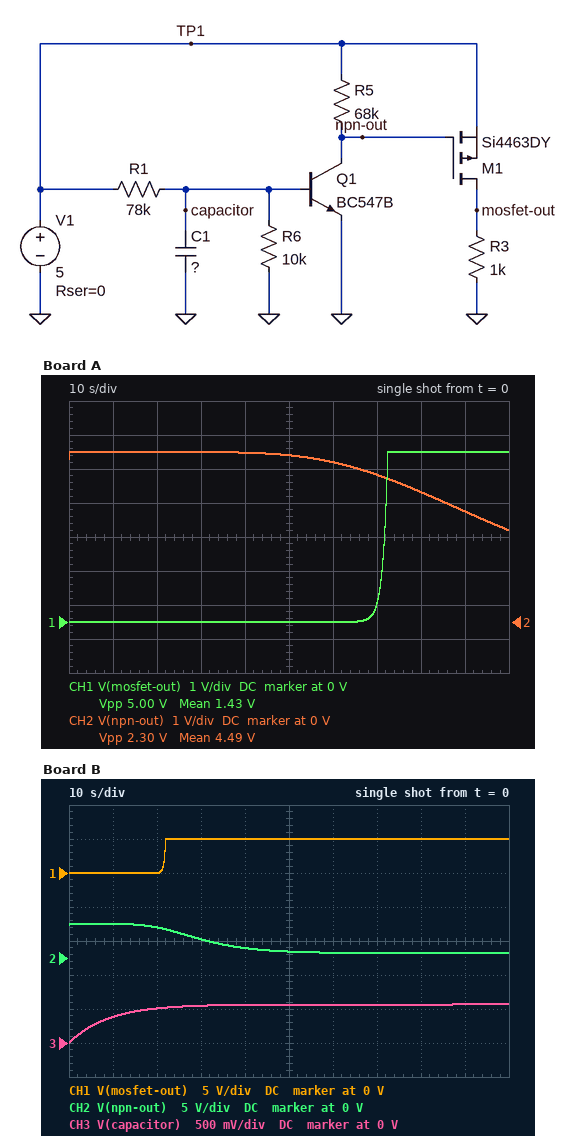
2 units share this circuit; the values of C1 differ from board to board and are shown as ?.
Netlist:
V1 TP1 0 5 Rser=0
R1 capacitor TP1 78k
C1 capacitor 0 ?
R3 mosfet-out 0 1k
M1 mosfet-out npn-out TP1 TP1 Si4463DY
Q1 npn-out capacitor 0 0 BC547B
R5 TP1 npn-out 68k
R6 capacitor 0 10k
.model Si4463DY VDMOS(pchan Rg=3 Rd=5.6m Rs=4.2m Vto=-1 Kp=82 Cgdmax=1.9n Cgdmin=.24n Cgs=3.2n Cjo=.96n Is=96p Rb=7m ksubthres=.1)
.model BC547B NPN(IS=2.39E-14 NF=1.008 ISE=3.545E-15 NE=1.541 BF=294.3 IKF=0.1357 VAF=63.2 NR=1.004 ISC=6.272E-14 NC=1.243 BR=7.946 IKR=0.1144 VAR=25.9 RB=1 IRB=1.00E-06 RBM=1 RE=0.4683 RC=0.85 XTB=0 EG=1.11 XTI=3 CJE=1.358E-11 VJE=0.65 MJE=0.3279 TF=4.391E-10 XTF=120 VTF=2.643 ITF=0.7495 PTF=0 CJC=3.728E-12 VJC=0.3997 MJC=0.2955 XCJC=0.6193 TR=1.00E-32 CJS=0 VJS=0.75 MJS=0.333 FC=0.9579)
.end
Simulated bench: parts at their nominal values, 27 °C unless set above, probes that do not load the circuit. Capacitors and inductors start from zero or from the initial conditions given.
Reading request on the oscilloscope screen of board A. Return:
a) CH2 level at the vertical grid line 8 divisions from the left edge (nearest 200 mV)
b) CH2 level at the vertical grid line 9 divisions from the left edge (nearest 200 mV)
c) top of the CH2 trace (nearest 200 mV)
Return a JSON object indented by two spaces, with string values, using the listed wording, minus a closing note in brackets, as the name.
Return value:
{
  "CH2 level at the vertical grid line 8 divisions from the left edge": "3.8 V",
  "CH2 level at the vertical grid line 9 divisions from the left edge": "3.2 V",
  "top of the CH2 trace": "5.0 V"
}
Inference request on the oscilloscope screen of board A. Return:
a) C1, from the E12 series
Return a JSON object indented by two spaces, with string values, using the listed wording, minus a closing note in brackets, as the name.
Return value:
{
  "C1, from the E12 series": "3.3 mF"
}
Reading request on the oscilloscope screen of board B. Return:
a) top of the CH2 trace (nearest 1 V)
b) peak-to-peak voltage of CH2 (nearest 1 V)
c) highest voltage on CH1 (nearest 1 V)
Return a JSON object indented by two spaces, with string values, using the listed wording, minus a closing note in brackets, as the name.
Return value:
{
  "top of the CH2 trace": "5 V",
  "peak-to-peak voltage of CH2": "4 V",
  "highest voltage on CH1": "5 V"
}
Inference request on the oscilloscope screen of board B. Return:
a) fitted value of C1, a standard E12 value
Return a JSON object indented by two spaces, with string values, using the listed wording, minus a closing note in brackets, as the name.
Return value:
{
  "fitted value of C1, a standard E12 value": "1 mF"
}
